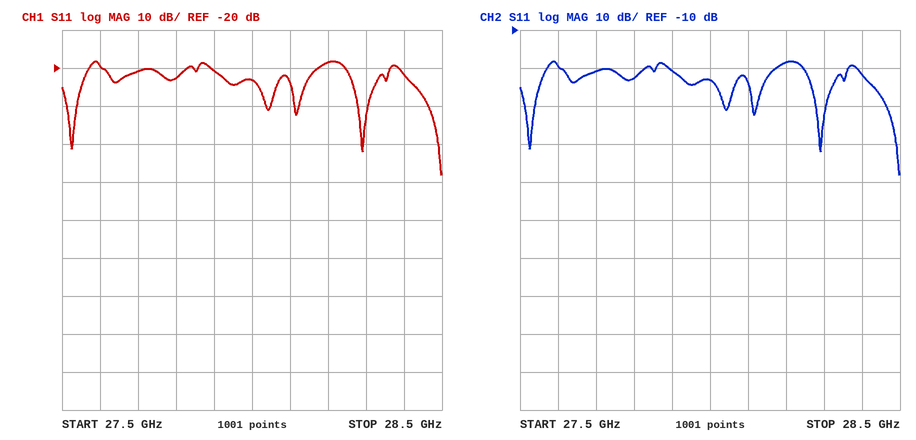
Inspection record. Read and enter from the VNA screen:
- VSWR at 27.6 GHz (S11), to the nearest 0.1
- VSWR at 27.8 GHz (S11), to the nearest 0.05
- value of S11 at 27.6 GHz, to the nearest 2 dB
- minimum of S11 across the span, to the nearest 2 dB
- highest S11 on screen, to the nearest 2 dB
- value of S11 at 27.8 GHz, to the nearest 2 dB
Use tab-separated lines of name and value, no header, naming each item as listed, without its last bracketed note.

VSWR at 27.6 GHz (S11), to the nearest 0.1	1.2
VSWR at 27.8 GHz (S11), to the nearest 0.05	1.15
value of S11 at 27.6 GHz, to the nearest 2 dB	-20 dB
minimum of S11 across the span, to the nearest 2 dB	-48 dB
highest S11 on screen, to the nearest 2 dB	-18 dB
value of S11 at 27.8 GHz, to the nearest 2 dB	-22 dB
